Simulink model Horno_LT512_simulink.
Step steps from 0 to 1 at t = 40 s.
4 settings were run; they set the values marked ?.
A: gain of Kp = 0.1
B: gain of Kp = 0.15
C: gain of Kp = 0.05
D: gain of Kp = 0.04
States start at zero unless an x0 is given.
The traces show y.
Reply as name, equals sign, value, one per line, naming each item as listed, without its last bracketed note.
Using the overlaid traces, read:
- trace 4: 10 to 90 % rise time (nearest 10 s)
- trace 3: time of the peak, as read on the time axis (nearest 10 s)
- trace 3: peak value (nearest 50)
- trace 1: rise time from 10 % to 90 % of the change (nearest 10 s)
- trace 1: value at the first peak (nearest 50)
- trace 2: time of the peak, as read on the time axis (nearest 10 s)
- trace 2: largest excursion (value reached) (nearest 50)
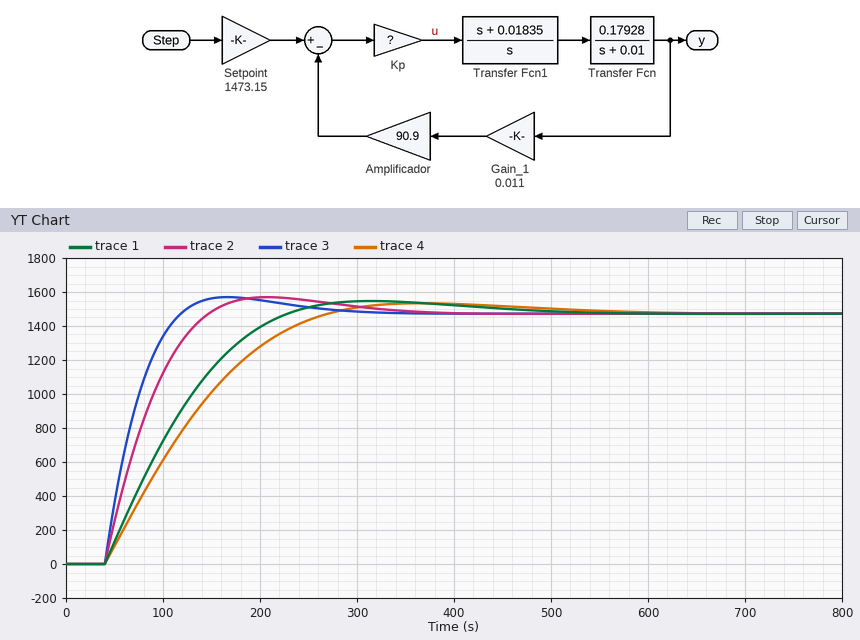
trace 4: 10 to 90 % rise time = 160 s
trace 3: time of the peak, as read on the time axis = 170 s
trace 3: peak value = 1550
trace 1: rise time from 10 % to 90 % of the change = 130 s
trace 1: value at the first peak = 1550
trace 2: time of the peak, as read on the time axis = 210 s
trace 2: largest excursion (value reached) = 1550
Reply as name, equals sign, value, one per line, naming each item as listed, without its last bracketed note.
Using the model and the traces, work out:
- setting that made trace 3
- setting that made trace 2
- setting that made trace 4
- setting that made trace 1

setting that made trace 3 = B
setting that made trace 2 = A
setting that made trace 4 = D
setting that made trace 1 = C
